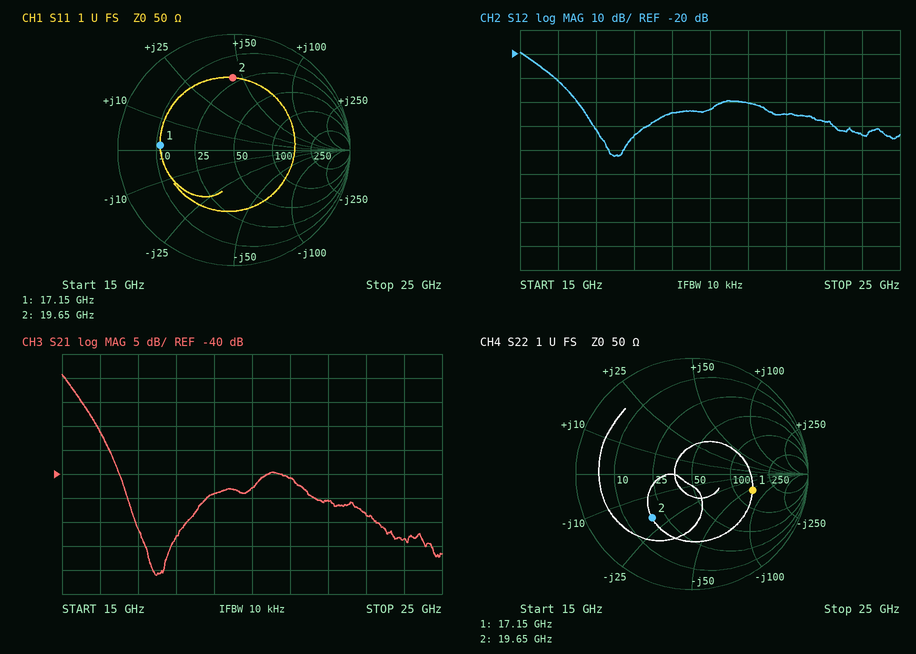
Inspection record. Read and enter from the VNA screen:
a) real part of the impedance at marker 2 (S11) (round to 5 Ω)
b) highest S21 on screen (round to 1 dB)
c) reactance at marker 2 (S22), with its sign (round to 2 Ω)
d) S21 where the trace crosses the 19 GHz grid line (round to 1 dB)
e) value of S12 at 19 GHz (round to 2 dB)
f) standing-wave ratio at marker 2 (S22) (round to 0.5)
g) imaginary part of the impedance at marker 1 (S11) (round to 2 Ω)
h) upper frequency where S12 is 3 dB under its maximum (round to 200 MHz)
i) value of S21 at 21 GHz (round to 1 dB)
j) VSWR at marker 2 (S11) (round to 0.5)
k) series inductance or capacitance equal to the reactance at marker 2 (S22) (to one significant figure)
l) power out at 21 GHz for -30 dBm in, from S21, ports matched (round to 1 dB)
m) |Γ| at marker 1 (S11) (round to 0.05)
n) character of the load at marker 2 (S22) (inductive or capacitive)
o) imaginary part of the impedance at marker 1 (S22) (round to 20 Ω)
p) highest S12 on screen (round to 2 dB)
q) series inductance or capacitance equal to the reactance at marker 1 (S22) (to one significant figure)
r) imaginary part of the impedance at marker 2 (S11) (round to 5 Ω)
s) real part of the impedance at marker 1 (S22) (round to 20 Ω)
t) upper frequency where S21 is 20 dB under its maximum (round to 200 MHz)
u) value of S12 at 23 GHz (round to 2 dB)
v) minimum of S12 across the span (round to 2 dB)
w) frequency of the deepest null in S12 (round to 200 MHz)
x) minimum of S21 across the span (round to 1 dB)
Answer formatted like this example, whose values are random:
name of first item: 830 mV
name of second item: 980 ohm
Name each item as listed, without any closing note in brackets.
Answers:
real part of the impedance at marker 2 (S11): 20 Ω
highest S21 on screen: -19 dB
reactance at marker 2 (S22), with its sign: -20 Ω
S21 where the trace crosses the 19 GHz grid line: -44 dB
value of S12 at 19 GHz: -44 dB
standing-wave ratio at marker 2 (S22): 3.0
imaginary part of the impedance at marker 1 (S11): +2 Ω
upper frequency where S12 is 3 dB under its maximum: 15.2 GHz
value of S21 at 21 GHz: -41 dB
VSWR at marker 2 (S11): 4.5
series inductance or capacitance equal to the reactance at marker 2 (S22): 400 fF
power out at 21 GHz for -30 dBm in, from S21, ports matched: -71 dBm
|Γ| at marker 1 (S11): 0.65
character of the load at marker 2 (S22): capacitive
imaginary part of the impedance at marker 1 (S22): -60 Ω
highest S12 on screen: -20 dB
series inductance or capacitance equal to the reactance at marker 1 (S22): 200 fF
imaginary part of the impedance at marker 2 (S11): +45 Ω
real part of the impedance at marker 1 (S22): 140 Ω
upper frequency where S21 is 20 dB under its maximum: 16.4 GHz
value of S12 at 23 GHz: -48 dB
minimum of S12 across the span: -62 dB
frequency of the deepest null in S12: 17.4 GHz
minimum of S21 across the span: -61 dB
